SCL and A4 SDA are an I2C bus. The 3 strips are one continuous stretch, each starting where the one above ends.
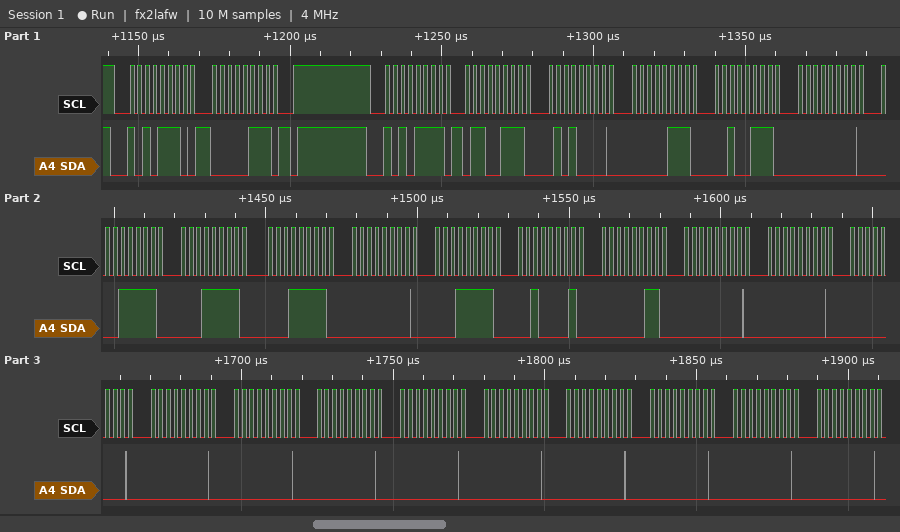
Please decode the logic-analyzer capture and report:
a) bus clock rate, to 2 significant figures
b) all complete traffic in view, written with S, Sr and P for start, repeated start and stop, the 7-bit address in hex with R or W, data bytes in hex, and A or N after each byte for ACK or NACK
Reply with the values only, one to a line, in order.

400 kHz
S 57W A 07 A P S 57R A 67 A 50 A 07 A 27 A 00 A 1F A 1F A 1F A 00 A 1F A 21 A 03 A 00 A 00 A 00 A 00 A 00 A 00 A 00 A 00 A 00 A 00 A 00 A 00 A
